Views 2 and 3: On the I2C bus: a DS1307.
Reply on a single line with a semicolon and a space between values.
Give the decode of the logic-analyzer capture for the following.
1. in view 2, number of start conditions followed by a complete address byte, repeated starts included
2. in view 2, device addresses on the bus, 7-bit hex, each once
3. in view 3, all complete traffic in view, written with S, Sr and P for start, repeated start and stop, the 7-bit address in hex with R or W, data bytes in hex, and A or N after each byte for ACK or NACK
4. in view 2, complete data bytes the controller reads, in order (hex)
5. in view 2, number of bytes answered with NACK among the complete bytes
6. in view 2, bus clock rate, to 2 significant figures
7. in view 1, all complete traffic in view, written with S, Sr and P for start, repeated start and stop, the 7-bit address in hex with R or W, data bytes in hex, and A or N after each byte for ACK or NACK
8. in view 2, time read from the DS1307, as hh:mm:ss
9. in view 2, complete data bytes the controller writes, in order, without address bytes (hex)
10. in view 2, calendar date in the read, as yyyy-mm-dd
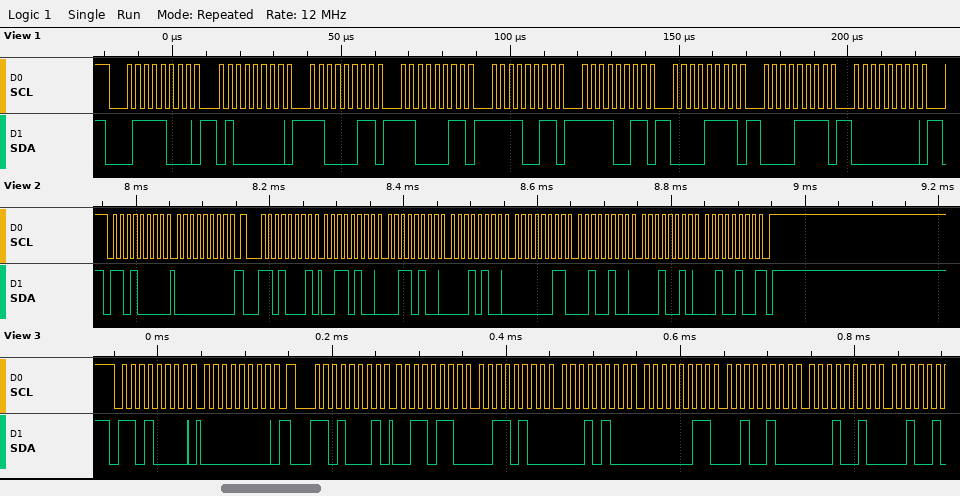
2; 0x68; S 68W A 00 A Sr 68R A 36 A 34 A 14 A 03 A 24 A 12 A; 34 34 14 03 24 12 24; 1; 100 kHz; S 3CW A 40 A C3 A C3 A F3 A F3 A 0F A 0F A 00 A; 14:34:34; 00; 2024-12-24
